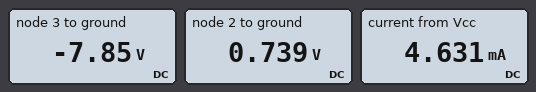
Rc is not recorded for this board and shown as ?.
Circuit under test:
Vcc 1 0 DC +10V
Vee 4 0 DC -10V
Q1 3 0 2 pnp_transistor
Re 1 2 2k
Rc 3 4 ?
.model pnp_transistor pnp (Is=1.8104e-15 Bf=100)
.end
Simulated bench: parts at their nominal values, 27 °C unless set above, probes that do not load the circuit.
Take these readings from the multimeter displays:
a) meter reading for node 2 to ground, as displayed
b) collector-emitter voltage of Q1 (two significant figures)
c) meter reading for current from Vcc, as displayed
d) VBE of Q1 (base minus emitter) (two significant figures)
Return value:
0.739 V
-8.6 V
4.631 mA
-740 mV
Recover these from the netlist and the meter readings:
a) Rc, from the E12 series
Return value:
470 Ω
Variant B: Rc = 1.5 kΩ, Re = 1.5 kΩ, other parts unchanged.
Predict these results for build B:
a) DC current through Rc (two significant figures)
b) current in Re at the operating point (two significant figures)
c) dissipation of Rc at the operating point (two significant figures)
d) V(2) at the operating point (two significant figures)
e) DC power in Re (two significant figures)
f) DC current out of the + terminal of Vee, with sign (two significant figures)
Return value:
6.1 mA
6.2 mA
56 mW
750 mV
57 mW
-6.1 mA
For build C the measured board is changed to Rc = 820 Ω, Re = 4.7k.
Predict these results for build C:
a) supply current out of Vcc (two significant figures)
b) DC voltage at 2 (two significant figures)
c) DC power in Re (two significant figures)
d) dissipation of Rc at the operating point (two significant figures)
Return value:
2.0 mA
720 mV
18 mW
3.1 mW
